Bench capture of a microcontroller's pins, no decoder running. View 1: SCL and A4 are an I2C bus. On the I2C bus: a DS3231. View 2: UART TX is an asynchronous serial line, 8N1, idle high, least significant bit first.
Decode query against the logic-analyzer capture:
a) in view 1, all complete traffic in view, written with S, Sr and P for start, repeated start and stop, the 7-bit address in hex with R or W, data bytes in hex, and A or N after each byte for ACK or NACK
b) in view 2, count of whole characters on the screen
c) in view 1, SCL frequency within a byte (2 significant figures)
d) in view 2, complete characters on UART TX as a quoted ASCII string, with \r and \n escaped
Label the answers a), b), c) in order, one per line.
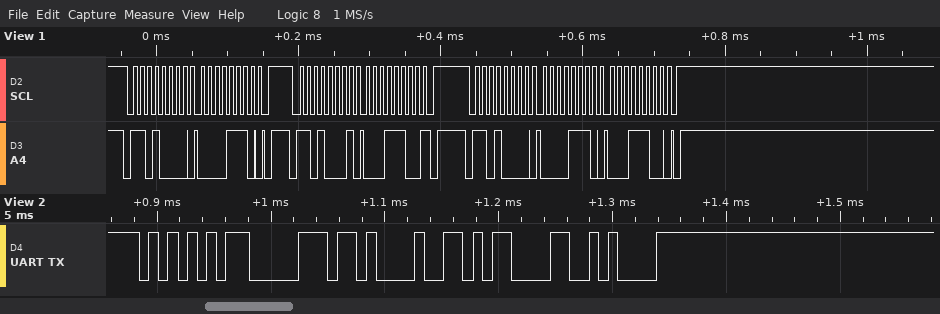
a) S 68W A 0E A P S 68R A 1C N P S 68W A 0E A 1C A P
b) 5
c) 100 kHz
d) "Up!\r\n"
